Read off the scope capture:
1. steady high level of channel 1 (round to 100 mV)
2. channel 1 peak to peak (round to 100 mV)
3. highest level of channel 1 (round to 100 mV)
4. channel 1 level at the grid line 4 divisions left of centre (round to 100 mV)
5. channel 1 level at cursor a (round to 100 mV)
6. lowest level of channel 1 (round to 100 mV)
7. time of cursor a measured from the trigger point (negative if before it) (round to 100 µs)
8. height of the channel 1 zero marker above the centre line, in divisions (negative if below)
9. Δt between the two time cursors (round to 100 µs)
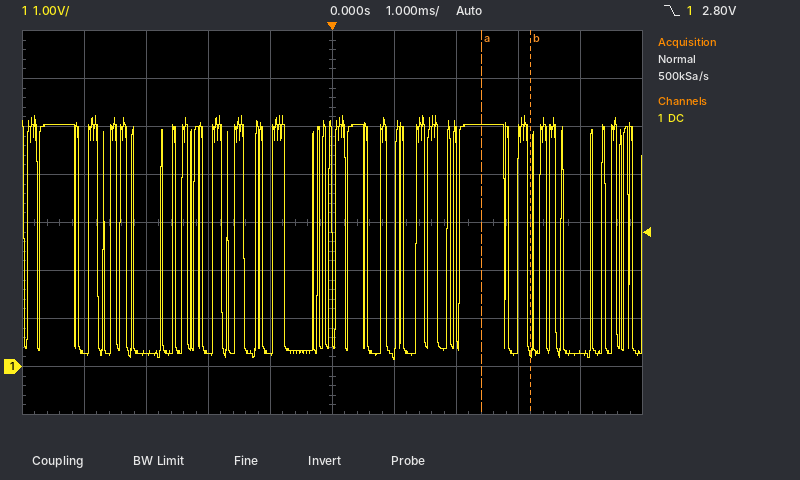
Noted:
5.0 V
5.1 V
5.2 V
300 mV
5.0 V
100 mV
+2.4 ms
-3.0 div
800 µs
